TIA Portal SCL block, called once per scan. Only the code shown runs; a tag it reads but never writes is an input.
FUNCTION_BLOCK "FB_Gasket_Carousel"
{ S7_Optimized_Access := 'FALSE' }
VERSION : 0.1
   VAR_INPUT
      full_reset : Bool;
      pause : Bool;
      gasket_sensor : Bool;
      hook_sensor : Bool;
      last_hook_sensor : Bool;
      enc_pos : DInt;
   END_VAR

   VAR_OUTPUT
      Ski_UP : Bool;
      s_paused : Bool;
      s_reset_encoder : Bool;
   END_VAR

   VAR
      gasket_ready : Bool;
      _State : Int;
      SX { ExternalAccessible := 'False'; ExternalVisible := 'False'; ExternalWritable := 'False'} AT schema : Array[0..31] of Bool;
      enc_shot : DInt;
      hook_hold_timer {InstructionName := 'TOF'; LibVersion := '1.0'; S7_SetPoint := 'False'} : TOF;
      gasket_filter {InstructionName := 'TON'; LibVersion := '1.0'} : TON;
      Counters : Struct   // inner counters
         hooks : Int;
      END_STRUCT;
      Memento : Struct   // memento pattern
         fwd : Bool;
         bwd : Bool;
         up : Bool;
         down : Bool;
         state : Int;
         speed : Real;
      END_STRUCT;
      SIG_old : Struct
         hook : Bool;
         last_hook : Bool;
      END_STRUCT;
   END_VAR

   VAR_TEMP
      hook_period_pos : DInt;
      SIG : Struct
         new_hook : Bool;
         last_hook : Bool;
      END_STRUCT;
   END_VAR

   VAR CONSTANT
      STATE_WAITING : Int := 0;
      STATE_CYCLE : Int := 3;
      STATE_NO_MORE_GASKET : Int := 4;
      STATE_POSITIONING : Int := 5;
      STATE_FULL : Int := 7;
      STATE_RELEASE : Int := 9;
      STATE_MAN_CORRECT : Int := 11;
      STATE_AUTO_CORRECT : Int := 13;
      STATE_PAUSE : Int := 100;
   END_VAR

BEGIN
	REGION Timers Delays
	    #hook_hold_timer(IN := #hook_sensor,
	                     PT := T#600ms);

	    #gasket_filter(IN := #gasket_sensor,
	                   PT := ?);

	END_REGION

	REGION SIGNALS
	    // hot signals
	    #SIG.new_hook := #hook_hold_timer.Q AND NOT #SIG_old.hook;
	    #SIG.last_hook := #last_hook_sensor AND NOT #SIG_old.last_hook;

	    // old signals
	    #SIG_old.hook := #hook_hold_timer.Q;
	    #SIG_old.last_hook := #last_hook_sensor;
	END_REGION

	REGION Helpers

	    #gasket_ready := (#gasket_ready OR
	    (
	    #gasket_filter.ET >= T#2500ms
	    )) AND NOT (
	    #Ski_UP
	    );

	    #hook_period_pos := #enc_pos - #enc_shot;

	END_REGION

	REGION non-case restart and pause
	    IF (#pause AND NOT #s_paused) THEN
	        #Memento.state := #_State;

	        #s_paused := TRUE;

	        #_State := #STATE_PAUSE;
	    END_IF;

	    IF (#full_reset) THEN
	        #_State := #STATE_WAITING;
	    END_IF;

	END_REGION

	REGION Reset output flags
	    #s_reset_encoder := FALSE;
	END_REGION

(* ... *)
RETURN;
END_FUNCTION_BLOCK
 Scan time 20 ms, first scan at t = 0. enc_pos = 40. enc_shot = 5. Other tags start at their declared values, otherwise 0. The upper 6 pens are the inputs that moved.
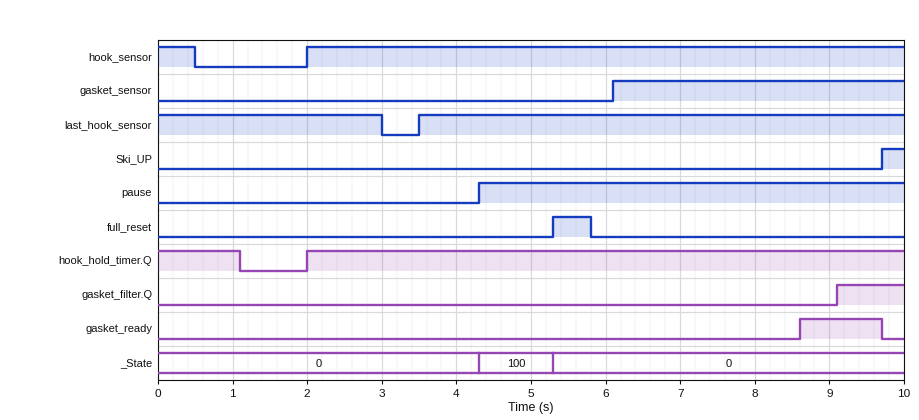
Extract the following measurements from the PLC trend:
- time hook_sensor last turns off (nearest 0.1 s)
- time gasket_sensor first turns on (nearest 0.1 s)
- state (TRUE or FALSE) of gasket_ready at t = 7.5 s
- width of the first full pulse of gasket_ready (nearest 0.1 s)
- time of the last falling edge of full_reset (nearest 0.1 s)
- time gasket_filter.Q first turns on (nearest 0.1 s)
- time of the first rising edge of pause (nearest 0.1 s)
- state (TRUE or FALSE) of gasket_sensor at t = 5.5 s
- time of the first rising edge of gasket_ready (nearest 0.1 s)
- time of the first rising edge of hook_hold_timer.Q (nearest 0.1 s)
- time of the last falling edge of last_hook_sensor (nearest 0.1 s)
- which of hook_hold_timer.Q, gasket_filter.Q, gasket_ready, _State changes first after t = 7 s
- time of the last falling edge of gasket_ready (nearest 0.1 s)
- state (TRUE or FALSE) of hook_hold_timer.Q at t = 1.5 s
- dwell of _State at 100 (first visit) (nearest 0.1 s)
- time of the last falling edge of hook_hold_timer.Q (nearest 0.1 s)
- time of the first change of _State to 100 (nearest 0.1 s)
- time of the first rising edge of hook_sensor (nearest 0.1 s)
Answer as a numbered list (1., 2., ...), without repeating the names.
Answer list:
1. 0.5 s
2. 6.1 s
3. FALSE
4. 1.1 s
5. 5.8 s
6. 9.1 s
7. 4.3 s
8. FALSE
9. 8.6 s
10. 2.0 s
11. 3.0 s
12. gasket_ready
13. 9.7 s
14. FALSE
15. 1.0 s
16. 1.1 s
17. 4.3 s
18. 2.0 s
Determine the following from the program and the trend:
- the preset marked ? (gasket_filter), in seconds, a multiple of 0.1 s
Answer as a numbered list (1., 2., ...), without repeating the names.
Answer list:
1. 3.0 s
